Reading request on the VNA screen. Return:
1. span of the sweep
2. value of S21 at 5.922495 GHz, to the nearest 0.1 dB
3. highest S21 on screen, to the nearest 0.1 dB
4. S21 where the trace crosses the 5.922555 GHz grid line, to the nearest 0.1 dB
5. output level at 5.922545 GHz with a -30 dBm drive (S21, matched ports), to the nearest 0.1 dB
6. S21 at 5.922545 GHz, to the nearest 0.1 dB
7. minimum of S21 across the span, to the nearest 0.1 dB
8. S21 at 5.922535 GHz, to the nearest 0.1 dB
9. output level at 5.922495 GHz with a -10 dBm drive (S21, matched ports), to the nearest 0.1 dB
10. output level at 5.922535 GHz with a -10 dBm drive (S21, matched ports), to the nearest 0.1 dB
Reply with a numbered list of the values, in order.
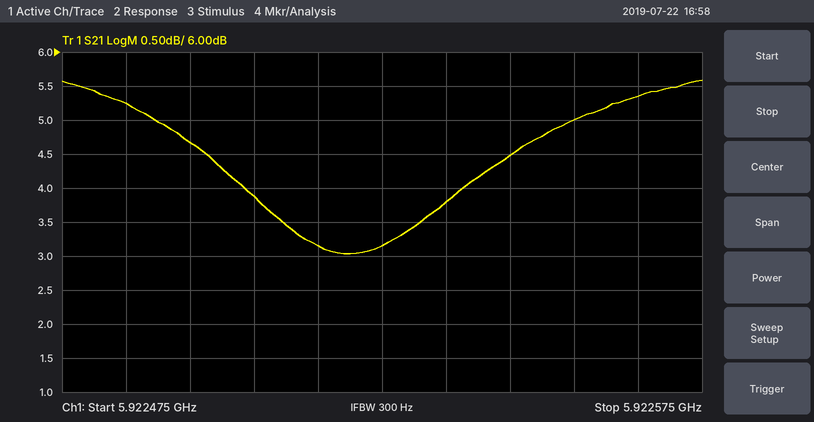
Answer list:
1. 100 kHz
2. 4.7 dB
3. 5.6 dB
4. 5.0 dB
5. -25.5 dBm
6. 4.5 dB
7. 3.0 dB
8. 3.8 dB
9. -5.3 dBm
10. -6.2 dBm
